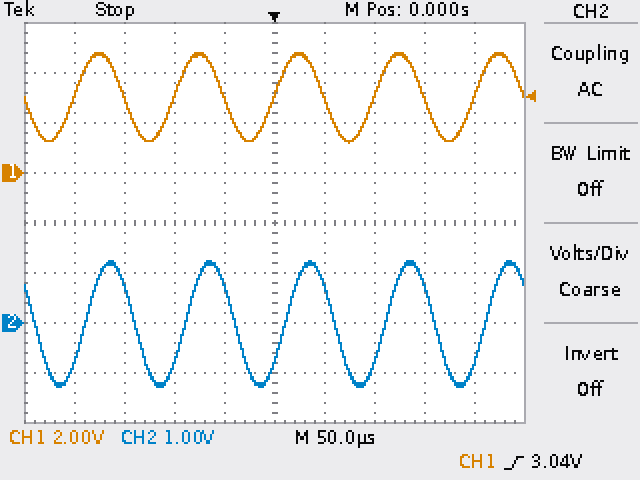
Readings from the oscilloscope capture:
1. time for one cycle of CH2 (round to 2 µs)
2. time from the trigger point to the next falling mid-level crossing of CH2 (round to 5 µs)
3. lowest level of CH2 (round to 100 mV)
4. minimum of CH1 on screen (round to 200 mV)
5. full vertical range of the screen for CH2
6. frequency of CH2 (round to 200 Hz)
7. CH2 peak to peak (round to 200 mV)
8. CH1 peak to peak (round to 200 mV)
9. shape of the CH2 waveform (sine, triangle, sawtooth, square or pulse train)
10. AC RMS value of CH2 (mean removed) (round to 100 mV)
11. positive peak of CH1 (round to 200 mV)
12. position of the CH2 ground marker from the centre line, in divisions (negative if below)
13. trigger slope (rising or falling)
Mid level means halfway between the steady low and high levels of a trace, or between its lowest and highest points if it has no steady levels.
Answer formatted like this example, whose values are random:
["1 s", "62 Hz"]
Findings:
["100 µs", "60 µs", "-1.3 V", "1.2 V", "8 V", "10.0 kHz", "2.6 V", "3.6 V", "sine", "900 mV", "4.8 V", "-2.0 div", "rising"]
